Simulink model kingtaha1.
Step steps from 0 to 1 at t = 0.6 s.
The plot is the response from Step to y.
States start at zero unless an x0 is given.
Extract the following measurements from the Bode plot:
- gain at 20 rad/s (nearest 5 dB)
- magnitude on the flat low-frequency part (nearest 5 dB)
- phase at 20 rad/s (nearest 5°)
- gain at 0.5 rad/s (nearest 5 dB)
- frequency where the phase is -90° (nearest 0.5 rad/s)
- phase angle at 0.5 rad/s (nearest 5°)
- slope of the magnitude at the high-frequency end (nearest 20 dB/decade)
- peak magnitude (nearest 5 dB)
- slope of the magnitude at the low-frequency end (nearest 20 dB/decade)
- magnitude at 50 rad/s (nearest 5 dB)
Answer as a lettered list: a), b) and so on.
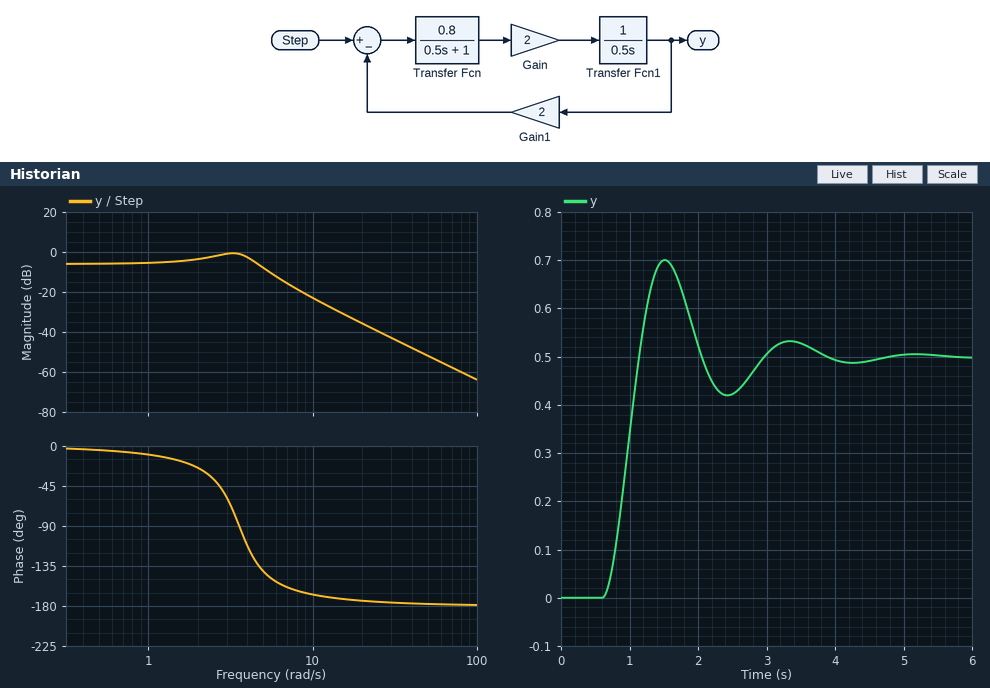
a) -35 dB
b) -5 dB
c) -175°
d) -5 dB
e) 3.5 rad/s
f) -5°
g) -40 dB/decade
h) 0 dB
i) 0 dB/decade
j) -50 dB
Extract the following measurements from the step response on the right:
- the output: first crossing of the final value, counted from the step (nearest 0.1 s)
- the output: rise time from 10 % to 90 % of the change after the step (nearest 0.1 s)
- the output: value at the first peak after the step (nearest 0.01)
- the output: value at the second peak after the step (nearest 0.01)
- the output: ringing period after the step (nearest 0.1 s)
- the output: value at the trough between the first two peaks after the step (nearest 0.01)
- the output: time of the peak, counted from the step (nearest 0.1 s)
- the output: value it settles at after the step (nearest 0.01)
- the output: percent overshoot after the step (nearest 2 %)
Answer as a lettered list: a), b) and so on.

a) 0.5 s
b) 0.4 s
c) 0.70
d) 0.53
e) 1.8 s
f) 0.42
g) 0.9 s
h) 0.50
i) 40 %
